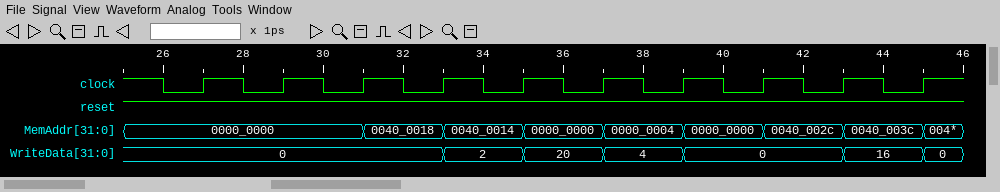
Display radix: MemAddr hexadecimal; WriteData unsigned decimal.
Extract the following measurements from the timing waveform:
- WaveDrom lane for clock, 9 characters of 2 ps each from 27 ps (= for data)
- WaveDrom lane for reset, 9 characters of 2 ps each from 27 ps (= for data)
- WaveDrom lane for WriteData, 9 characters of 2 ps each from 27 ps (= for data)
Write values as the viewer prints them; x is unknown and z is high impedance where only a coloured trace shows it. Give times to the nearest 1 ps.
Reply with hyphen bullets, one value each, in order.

- {name: 'clock', wave: 'p........'}
- {name: 'reset', wave: '1........'}
- {name: 'WriteData', wave: '=..====.=', data: '0 2 20 4 0 16'}
